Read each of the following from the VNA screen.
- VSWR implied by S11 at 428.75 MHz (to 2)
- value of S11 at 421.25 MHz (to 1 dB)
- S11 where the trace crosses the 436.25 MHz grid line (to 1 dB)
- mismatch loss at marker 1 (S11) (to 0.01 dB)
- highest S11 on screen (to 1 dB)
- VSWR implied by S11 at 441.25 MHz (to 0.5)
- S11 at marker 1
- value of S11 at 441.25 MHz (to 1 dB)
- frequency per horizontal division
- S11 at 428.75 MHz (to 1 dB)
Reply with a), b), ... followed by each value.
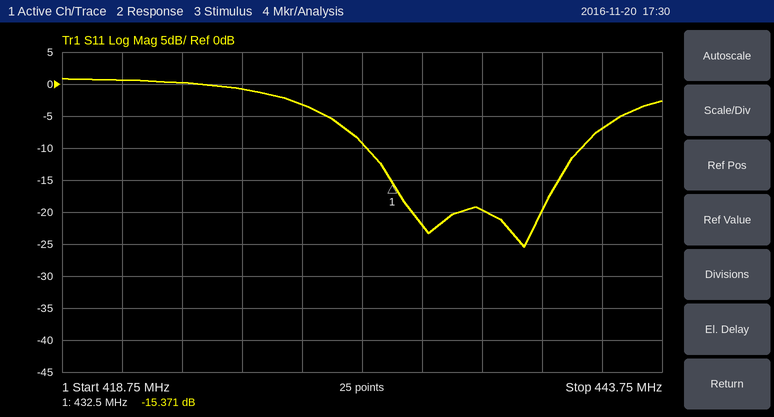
a) 6
b) 1 dB
c) -20 dB
d) 0.13 dB
e) 1 dB
f) 2.5
g) -15.371 dB
h) -7 dB
i) 2.5 MHz
j) -3 dB
